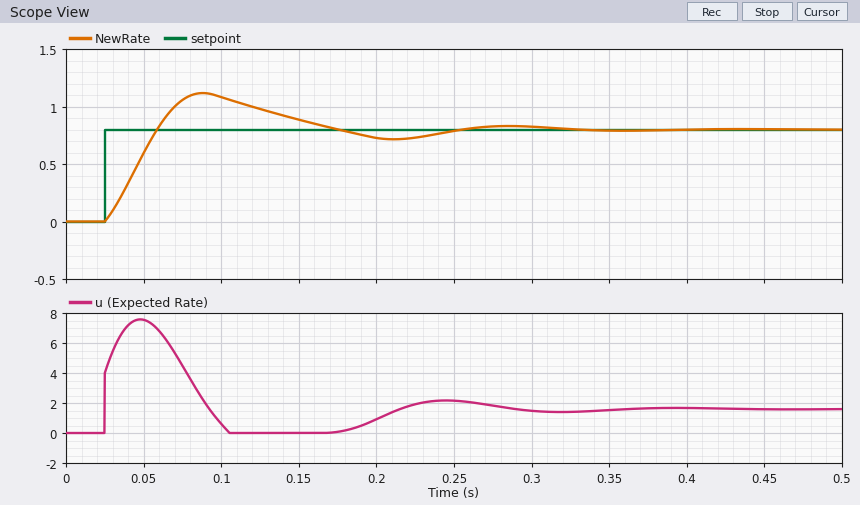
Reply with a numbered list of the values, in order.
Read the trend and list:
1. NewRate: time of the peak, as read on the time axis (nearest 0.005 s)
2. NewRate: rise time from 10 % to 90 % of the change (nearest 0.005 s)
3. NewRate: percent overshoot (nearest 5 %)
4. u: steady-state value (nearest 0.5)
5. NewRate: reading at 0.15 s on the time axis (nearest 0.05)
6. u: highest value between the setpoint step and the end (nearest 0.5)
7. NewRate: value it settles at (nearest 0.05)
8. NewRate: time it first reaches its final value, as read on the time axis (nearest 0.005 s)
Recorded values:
1. 0.090 s
2. 0.025 s
3. 40 %
4. 1.5
5. 0.90
6. 7.5
7. 0.80
8. 0.060 s
